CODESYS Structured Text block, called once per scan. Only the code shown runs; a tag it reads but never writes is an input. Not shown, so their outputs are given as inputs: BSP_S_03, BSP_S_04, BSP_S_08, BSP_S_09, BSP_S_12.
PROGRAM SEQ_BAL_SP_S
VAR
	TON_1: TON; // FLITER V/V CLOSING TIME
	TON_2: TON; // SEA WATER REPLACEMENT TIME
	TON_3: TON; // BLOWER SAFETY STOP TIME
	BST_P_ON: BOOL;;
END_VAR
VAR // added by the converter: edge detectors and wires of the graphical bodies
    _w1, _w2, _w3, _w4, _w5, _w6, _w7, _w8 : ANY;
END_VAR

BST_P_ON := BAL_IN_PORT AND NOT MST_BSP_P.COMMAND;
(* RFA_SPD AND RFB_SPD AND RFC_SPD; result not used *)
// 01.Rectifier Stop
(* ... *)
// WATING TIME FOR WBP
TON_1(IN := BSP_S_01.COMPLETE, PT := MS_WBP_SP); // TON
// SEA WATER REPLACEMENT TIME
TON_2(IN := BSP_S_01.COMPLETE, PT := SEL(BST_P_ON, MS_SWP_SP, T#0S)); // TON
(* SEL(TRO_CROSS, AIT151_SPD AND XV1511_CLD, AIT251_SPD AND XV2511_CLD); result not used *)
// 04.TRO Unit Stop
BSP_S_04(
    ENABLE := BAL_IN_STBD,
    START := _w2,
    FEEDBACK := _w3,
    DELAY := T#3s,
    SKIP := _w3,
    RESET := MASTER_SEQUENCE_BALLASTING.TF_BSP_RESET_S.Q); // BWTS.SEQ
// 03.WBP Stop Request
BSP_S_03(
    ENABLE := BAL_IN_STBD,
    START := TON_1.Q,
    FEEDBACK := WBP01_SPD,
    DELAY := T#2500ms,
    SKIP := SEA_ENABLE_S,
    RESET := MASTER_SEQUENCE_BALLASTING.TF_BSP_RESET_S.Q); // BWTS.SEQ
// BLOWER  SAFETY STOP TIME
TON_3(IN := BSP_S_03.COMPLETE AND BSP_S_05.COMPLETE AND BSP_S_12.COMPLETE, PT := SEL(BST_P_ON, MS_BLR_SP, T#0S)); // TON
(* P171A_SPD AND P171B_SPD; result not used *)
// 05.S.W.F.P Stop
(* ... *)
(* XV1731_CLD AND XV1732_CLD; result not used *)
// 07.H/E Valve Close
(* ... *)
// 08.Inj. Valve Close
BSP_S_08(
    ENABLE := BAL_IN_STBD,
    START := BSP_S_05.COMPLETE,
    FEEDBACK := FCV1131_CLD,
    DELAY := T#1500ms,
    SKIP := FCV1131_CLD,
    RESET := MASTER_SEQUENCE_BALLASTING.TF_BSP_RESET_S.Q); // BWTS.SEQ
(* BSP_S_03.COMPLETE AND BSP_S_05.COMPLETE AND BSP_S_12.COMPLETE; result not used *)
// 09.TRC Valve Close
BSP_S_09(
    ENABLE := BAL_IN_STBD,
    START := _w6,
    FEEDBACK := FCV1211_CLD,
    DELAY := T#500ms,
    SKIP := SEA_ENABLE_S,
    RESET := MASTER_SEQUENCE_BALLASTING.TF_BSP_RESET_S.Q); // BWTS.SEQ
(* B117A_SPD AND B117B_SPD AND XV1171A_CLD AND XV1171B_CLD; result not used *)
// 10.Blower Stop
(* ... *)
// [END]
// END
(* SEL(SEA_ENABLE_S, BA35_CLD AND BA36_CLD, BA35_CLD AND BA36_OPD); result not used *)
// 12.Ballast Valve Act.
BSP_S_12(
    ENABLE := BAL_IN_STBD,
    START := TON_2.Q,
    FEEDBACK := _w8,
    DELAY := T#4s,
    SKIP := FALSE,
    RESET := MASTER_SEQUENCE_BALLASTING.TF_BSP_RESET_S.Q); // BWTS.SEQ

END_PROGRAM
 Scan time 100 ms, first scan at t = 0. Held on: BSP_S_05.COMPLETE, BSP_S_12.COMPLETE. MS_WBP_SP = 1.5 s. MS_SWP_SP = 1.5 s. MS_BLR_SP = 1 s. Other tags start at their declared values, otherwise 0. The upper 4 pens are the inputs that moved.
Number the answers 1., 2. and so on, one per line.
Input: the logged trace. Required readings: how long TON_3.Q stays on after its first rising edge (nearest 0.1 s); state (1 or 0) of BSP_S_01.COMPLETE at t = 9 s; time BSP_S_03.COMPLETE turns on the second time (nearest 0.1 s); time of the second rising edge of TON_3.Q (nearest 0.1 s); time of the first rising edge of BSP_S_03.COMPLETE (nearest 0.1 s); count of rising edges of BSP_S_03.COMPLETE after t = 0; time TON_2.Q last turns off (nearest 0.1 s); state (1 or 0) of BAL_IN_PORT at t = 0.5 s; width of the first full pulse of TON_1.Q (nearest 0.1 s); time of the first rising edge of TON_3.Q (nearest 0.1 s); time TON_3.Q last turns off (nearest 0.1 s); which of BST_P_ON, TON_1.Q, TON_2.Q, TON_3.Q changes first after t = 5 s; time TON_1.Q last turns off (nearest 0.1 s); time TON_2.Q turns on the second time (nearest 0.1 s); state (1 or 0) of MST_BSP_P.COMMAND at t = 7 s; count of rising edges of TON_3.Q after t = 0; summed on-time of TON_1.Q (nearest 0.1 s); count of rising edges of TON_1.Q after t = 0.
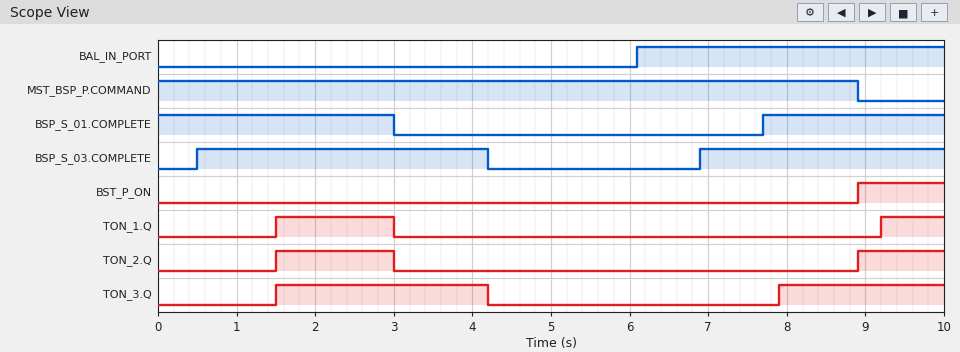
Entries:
1. 2.7 s
2. 1
3. 6.9 s
4. 7.9 s
5. 0.5 s
6. 2
7. 3.0 s
8. 0
9. 1.5 s
10. 1.5 s
11. 4.2 s
12. TON_3.Q
13. 3.0 s
14. 8.9 s
15. 1
16. 2
17. 2.3 s
18. 2
